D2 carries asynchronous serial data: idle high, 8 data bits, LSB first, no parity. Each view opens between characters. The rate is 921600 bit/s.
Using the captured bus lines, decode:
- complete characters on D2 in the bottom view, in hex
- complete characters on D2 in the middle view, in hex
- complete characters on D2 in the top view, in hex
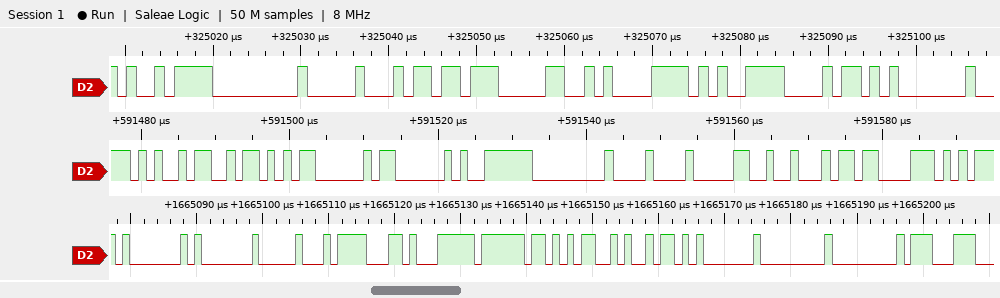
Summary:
01, 01, 10, 8F, F1, BF, 35, 69, 01, 00, 00, C7
A5, 5A, 03, 03, F9, 00, 08, 30, A2, C3
E9, 00, 10, DB, 30, E1, E5, 68, 01
